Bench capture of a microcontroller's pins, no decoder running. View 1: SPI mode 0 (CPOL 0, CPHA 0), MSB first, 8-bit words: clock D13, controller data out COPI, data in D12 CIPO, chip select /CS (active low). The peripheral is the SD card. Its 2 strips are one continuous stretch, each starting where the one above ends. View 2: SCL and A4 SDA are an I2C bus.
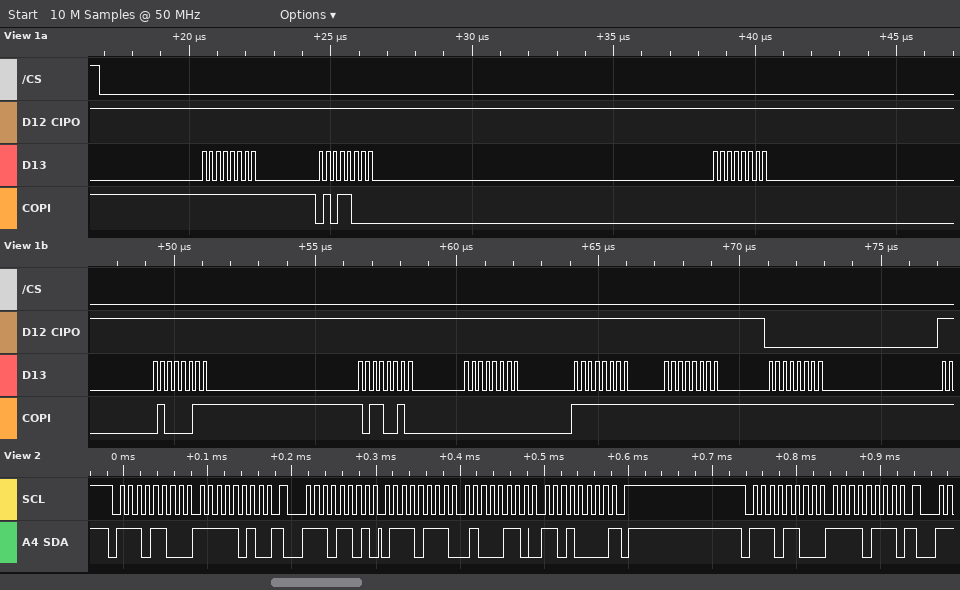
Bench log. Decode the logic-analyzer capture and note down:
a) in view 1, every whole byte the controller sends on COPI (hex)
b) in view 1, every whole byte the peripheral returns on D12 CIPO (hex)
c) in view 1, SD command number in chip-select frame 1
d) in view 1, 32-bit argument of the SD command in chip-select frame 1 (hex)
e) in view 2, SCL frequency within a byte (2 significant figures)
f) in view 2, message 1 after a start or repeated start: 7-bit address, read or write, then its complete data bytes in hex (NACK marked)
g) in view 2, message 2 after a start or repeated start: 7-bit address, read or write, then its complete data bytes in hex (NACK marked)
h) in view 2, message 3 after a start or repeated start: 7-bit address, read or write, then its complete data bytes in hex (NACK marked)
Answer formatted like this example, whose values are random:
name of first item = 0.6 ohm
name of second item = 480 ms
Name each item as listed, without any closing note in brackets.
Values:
in view 1, every whole byte the controller sends on COPI = 0xFF 0x58 0x00 0x43 0xB2 0x00 0xFF 0xFF 0xFF
in view 1, every whole byte the peripheral returns on D12 CIPO = 0xFF 0xFF 0xFF 0xFF 0xFF 0xFF 0xFF 0xFF 0x00
in view 1, SD command number in chip-select frame 1 = CMD24
in view 1, 32-bit argument of the SD command in chip-select frame 1 = 0x0043B200
in view 2, SCL frequency within a byte = 100 kHz
in view 2, message 1 after a start or repeated start: 7-bit address, read or write, then its complete data bytes in hex = 0x76 write: FA
in view 2, message 2 after a start or repeated start: 7-bit address, read or write, then its complete data bytes in hex = 0x76 read: 77 46 D0 NACK
in view 2, message 3 after a start or repeated start: 7-bit address, read or write, then its complete data bytes in hex = 0x76 write: F7
